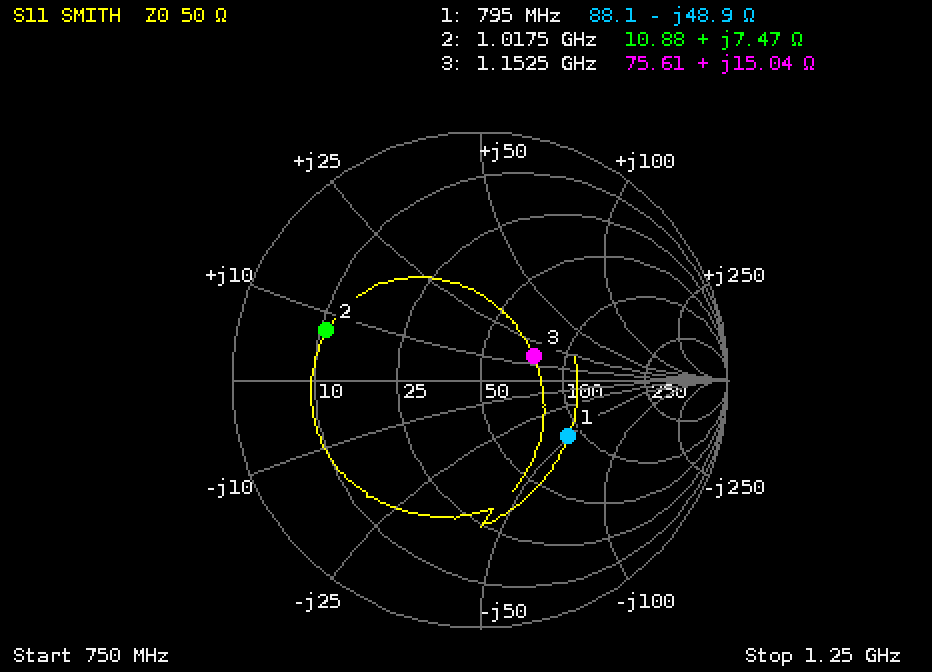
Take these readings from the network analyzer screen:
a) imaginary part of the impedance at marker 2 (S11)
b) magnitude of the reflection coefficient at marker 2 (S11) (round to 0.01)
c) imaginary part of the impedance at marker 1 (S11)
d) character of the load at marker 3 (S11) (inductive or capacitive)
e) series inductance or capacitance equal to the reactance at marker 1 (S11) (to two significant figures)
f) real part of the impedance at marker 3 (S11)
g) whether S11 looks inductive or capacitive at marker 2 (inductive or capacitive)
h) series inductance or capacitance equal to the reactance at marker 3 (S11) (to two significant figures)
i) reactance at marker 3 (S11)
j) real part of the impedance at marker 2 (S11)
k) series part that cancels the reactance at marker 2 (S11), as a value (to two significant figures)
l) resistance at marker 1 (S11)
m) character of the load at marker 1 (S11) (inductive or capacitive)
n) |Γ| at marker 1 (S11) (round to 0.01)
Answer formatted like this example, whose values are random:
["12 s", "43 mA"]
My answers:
["+7.47 Ω", "0.65", "-48.9 Ω", "inductive", "4.1 pF", "75.61 Ω", "inductive", "2.1 nH", "+15.04 Ω", "10.88 Ω", "21 pF", "88.1 Ω", "capacitive", "0.42"]
